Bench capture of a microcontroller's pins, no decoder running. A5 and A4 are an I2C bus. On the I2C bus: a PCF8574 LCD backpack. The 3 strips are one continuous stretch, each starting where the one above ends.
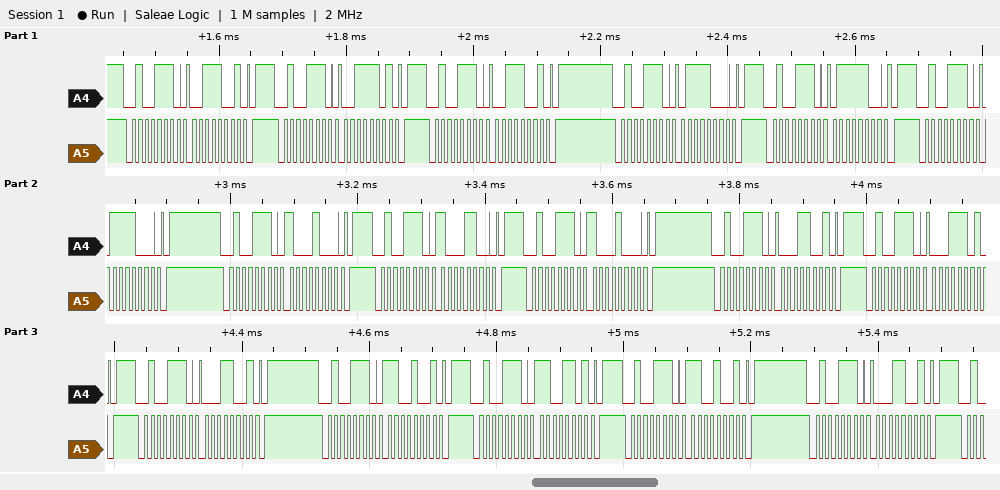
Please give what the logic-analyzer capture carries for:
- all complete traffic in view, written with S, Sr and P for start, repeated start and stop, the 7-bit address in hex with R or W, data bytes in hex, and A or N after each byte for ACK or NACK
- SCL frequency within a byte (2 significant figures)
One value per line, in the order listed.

S 27W A 39 A P S 27W A 3D A P S 27W A 39 A P S 27W A 78 A P S 27W A 7C A P S 27W A 78 A P S 27W A 88 A P S 27W A 8C A P S 27W A 88 A P S 27W A 19 A P S 27W A 1D A P S 27W A 19 A P S 27W A C9 A P S 27W A CD A P S 27W A C9 A P S 27W A 19 A P
100 kHz
